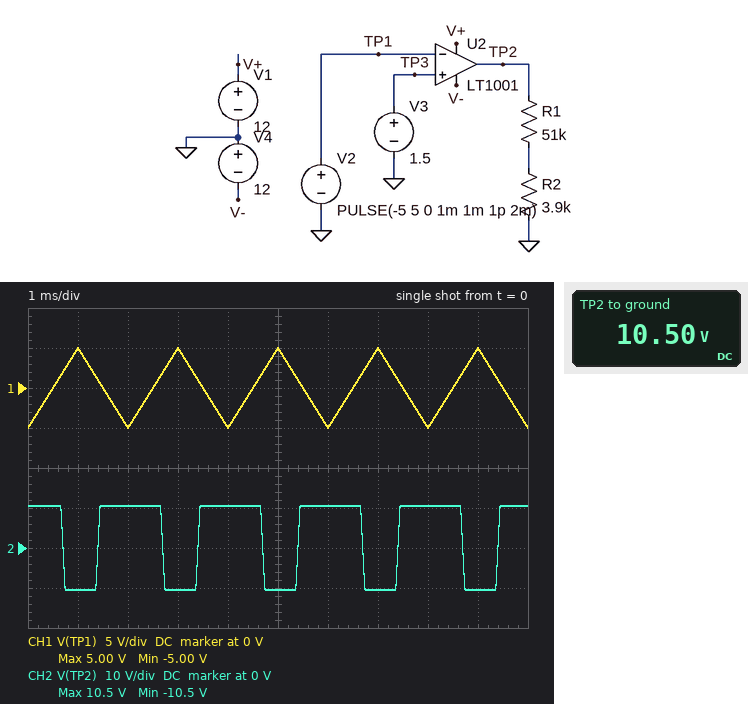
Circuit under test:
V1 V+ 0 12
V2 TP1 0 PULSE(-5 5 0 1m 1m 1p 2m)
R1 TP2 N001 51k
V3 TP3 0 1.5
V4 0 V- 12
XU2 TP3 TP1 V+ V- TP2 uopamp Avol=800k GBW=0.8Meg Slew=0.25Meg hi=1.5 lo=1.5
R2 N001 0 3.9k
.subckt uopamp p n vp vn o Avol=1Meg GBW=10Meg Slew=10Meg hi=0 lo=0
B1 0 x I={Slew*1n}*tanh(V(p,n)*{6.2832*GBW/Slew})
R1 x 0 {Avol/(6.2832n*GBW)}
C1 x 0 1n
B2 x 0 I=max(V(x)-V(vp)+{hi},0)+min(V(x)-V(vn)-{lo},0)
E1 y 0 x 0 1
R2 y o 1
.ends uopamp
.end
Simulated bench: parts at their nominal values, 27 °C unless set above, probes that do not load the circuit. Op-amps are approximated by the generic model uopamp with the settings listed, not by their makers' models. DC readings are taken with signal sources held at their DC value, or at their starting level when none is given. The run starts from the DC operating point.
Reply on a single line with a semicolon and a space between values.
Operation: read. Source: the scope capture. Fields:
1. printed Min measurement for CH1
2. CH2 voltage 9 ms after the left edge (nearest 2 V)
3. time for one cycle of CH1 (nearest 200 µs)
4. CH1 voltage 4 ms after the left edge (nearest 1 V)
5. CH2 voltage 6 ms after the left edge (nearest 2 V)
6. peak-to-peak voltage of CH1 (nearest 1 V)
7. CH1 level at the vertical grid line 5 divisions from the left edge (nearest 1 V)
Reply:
-5.00 V; -10 V; 2.0 ms; -5 V; 10 V; 10 V; 5 V
